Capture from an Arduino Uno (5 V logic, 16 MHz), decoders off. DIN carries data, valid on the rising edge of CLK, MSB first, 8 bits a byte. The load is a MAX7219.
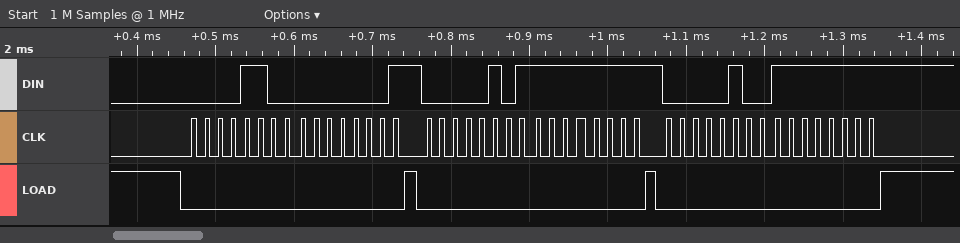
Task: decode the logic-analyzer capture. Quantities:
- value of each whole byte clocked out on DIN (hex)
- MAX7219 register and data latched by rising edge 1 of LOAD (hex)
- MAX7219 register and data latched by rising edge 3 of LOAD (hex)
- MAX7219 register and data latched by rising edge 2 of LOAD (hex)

0C 01 05 FF 04 FF
register 0xC, data 0x01
register 0x4, data 0xFF
register 0x5, data 0xFF
